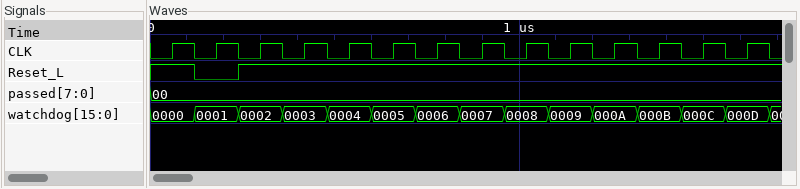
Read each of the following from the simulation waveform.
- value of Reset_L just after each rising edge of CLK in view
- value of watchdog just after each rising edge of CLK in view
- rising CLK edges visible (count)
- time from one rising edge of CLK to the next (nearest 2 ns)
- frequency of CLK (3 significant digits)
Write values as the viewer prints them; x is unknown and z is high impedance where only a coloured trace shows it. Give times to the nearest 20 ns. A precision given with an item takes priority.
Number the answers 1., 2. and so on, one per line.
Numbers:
1. 1 0 1 1 1 1 1 1 1 1 1 1 1 1
2. 0000, 0001, 0002, 0003, 0004, 0005, 0006, 0007, 0008, 0009, 000A, 000B, 000C, 000D
3. 14
4. 120 ns
5. 8.33 MHz
